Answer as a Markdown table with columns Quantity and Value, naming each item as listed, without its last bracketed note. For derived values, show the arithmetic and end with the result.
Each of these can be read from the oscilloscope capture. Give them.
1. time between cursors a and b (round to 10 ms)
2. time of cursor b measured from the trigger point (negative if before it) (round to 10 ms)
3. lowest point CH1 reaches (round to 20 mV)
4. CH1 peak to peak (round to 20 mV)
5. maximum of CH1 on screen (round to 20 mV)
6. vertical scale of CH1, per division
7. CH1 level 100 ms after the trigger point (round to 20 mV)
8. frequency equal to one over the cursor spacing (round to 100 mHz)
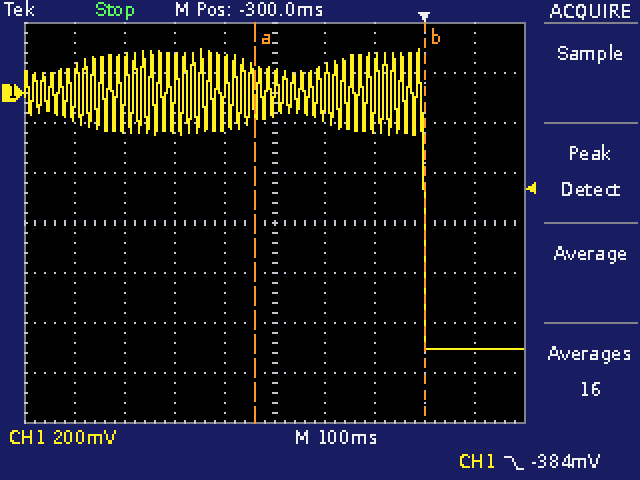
| Quantity | Value |
|---|---|
| time between cursors a and b | 340 ms |
| time of cursor b measured from the trigger point (negative if before it) | 0 ms |
| lowest point CH1 reaches | -1.02 V |
| CH1 peak to peak | 180 mV − (-1.02 V) = 1.20 V |
| maximum of CH1 on screen | 180 mV |
| vertical scale of CH1, per division | 200 mV |
| CH1 level 100 ms after the trigger point | -1.02 V |
| frequency equal to one over the cursor spacing | 1 / 340 ms ≈ 2.9 Hz |
